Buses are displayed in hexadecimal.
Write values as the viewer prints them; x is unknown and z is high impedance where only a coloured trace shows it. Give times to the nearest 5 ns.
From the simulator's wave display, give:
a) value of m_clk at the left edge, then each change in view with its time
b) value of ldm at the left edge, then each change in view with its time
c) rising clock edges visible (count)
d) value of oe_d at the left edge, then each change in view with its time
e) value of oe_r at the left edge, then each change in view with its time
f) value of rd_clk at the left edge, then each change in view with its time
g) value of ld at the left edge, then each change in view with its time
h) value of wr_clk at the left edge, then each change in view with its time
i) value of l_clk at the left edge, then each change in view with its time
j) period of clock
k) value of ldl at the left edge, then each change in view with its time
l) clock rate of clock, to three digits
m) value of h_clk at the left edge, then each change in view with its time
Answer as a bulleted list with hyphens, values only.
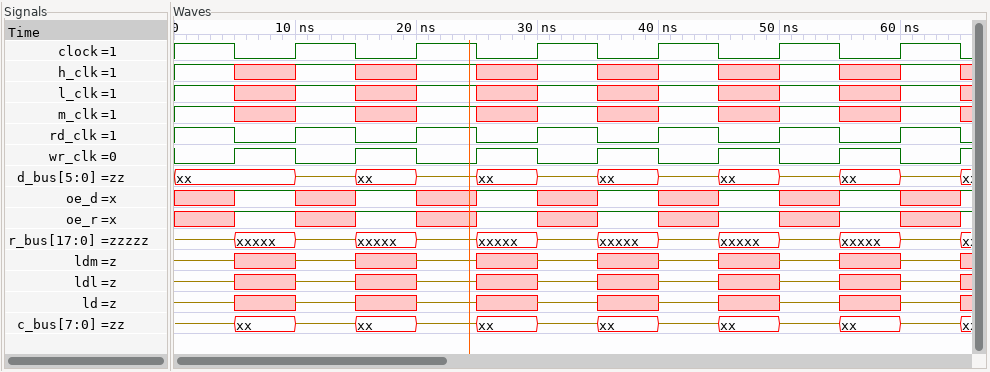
- 1, x at 5 ns, 1 at 10 ns, x at 15 ns, 1 at 20 ns, x at 25 ns, 1 at 30 ns, x at 35 ns, 1 at 40 ns, x at 45 ns, 1 at 50 ns, x at 55 ns, 1 at 60 ns, x at 65 ns
- z, x at 5 ns, z at 10 ns, x at 15 ns, z at 20 ns, x at 25 ns, z at 30 ns, x at 35 ns, z at 40 ns, x at 45 ns, z at 50 ns, x at 55 ns, z at 60 ns, x at 65 ns
- 6
- x, 1 at 5 ns, x at 10 ns, 1 at 15 ns, x at 20 ns, 1 at 25 ns, x at 30 ns, 1 at 35 ns, x at 40 ns, 1 at 45 ns, x at 50 ns, 1 at 55 ns, x at 60 ns, 1 at 65 ns
- x, 1 at 5 ns, x at 10 ns, 1 at 15 ns, x at 20 ns, 1 at 25 ns, x at 30 ns, 1 at 35 ns, x at 40 ns, 1 at 45 ns, x at 50 ns, 1 at 55 ns, x at 60 ns, 1 at 65 ns
- 1, 0 at 5 ns, 1 at 10 ns, 0 at 15 ns, 1 at 20 ns, 0 at 25 ns, 1 at 30 ns, 0 at 35 ns, 1 at 40 ns, 0 at 45 ns, 1 at 50 ns, 0 at 55 ns, 1 at 60 ns, 0 at 65 ns
- z, x at 5 ns, z at 10 ns, x at 15 ns, z at 20 ns, x at 25 ns, z at 30 ns, x at 35 ns, z at 40 ns, x at 45 ns, z at 50 ns, x at 55 ns, z at 60 ns, x at 65 ns
- 0, 1 at 5 ns, 0 at 10 ns, 1 at 15 ns, 0 at 20 ns, 1 at 25 ns, 0 at 30 ns, 1 at 35 ns, 0 at 40 ns, 1 at 45 ns, 0 at 50 ns, 1 at 55 ns, 0 at 60 ns, 1 at 65 ns
- 1, x at 5 ns, 1 at 10 ns, x at 15 ns, 1 at 20 ns, x at 25 ns, 1 at 30 ns, x at 35 ns, 1 at 40 ns, x at 45 ns, 1 at 50 ns, x at 55 ns, 1 at 60 ns, x at 65 ns
- 10 ns
- z, x at 5 ns, z at 10 ns, x at 15 ns, z at 20 ns, x at 25 ns, z at 30 ns, x at 35 ns, z at 40 ns, x at 45 ns, z at 50 ns, x at 55 ns, z at 60 ns, x at 65 ns
- 100 MHz
- 1, x at 5 ns, 1 at 10 ns, x at 15 ns, 1 at 20 ns, x at 25 ns, 1 at 30 ns, x at 35 ns, 1 at 40 ns, x at 45 ns, 1 at 50 ns, x at 55 ns, 1 at 60 ns, x at 65 ns
